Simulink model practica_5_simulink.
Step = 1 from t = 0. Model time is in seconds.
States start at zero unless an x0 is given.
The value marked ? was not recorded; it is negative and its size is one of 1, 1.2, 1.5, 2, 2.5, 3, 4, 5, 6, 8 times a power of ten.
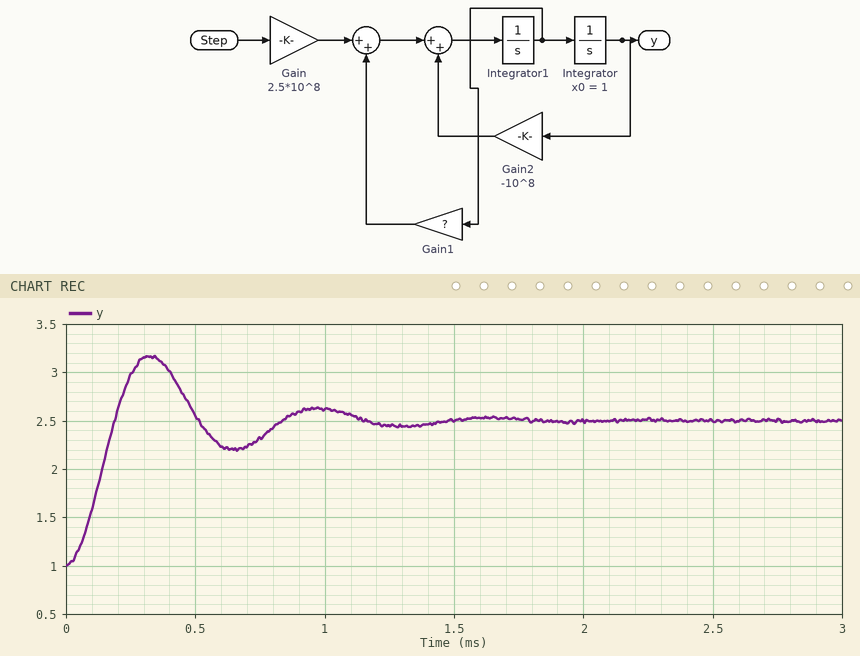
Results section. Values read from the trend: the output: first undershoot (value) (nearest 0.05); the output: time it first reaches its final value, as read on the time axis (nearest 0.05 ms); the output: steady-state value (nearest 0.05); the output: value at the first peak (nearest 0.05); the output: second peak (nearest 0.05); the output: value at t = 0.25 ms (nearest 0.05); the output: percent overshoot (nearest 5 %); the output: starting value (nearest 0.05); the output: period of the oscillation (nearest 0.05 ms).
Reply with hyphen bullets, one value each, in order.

- 2.20
- 0.20 ms
- 2.50
- 3.15
- 2.65
- 2.95
- 45 %
- 1.00
- 0.65 ms
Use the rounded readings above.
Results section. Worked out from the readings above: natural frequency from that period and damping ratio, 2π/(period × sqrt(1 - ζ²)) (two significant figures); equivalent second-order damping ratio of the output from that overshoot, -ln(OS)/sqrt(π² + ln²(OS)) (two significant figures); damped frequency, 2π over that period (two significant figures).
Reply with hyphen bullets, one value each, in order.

- 10.0 rad/ms
- 0.25
- 9.7 rad/ms
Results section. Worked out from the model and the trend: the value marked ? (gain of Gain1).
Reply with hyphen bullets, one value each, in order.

- -5000
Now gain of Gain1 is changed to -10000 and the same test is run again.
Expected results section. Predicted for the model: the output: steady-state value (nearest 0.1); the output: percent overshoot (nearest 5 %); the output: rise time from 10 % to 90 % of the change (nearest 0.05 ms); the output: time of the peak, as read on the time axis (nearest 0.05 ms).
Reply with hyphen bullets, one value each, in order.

- 2.5
- 15 %
- 0.15 ms
- 0.35 ms
